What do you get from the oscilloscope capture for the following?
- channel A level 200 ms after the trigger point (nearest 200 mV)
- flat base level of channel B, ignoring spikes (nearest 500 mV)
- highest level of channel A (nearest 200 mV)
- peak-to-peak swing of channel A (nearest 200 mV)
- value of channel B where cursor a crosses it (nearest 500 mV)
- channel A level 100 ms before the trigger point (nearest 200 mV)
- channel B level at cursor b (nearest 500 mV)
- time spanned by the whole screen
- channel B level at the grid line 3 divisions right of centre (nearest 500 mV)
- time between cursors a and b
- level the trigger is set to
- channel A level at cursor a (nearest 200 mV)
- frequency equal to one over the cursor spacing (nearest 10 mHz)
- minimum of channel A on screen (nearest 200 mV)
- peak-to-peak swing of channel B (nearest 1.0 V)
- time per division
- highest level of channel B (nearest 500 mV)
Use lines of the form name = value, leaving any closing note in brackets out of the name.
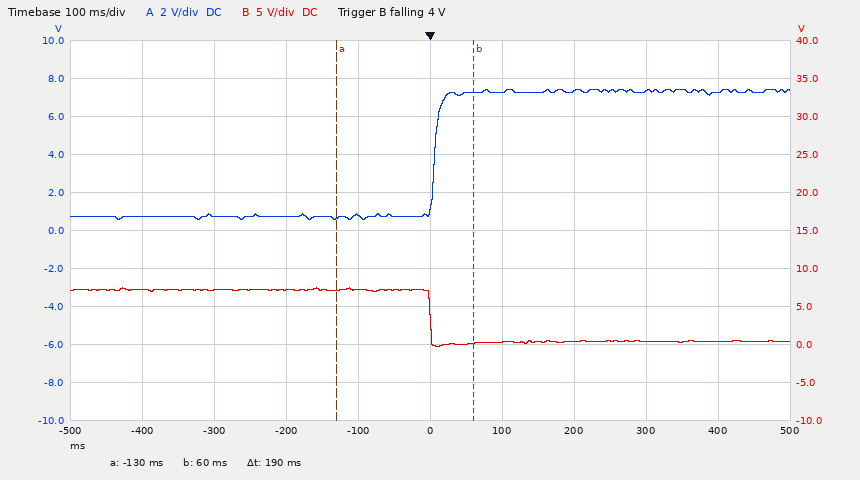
channel A level 200 ms after the trigger point = 7.4 V
flat base level of channel B, ignoring spikes = 500 mV
highest level of channel A = 7.4 V
peak-to-peak swing of channel A = 6.8 V
value of channel B where cursor a crosses it = 7.0 V
channel A level 100 ms before the trigger point = 800 mV
channel B level at cursor b = 0.0 V
time spanned by the whole screen = 1 s
channel B level at the grid line 3 divisions right of centre = 500 mV
time between cursors a and b = 190 ms
level the trigger is set to = 4 V
channel A level at cursor a = 600 mV
frequency equal to one over the cursor spacing = 5.26 Hz
minimum of channel A on screen = 600 mV
peak-to-peak swing of channel B = 8.0 V
time per division = 100 ms
highest level of channel B = 7.5 V
